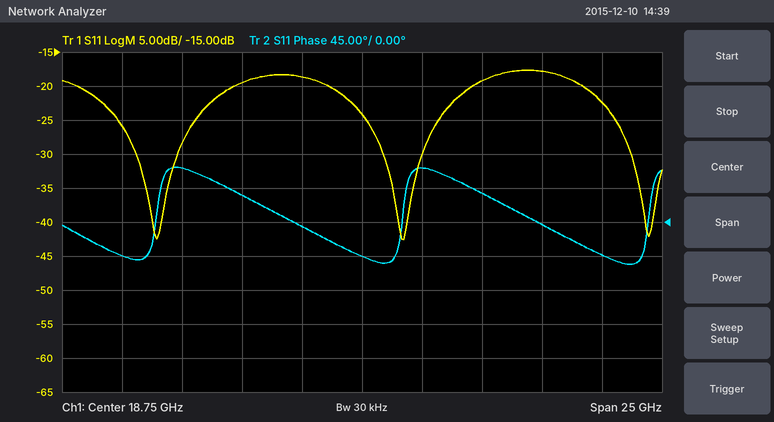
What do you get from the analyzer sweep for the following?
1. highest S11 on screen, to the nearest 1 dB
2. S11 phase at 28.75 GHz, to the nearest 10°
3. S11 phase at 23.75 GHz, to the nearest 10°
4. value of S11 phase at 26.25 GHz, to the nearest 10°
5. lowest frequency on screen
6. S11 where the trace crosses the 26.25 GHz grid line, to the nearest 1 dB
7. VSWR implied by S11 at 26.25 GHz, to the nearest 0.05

-18 dB
-40°
40°
0°
6.25 GHz
-18 dB
1.30
